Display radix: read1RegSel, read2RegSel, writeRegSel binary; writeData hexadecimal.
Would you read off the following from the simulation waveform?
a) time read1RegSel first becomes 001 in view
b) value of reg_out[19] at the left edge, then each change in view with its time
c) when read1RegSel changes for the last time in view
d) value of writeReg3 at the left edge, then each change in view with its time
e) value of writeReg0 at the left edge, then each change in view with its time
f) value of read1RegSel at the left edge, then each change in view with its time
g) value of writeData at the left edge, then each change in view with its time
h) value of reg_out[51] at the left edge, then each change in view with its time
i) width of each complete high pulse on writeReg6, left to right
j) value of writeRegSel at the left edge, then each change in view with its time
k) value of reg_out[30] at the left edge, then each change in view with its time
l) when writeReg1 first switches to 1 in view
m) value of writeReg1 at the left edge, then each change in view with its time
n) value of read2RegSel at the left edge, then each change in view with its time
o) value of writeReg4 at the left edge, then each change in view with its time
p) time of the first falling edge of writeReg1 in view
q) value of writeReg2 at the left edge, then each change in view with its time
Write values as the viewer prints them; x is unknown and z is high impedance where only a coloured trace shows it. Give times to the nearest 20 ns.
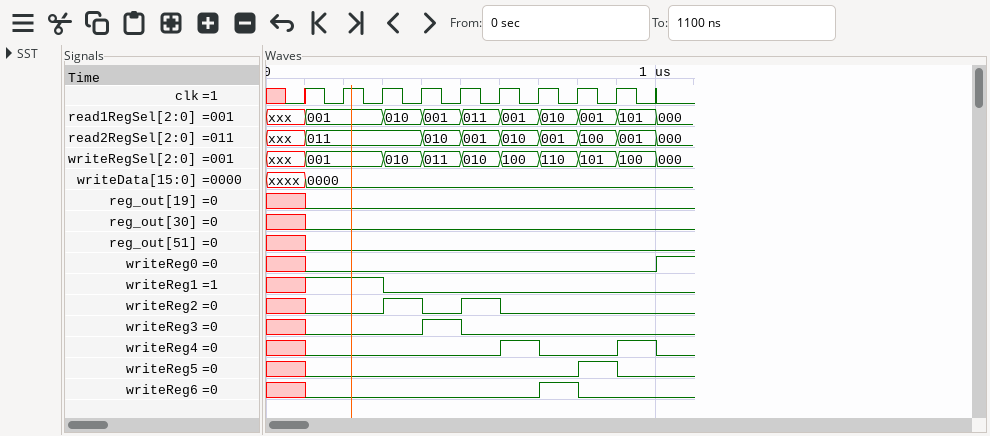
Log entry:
100 ns
x, 0 at 100 ns
1000 ns
x, 0 at 100 ns, 1 at 400 ns, 0 at 500 ns
x, 0 at 100 ns, 1 at 1000 ns
xxx, 001 at 100 ns, 010 at 300 ns, 001 at 400 ns, 011 at 500 ns, 001 at 600 ns, 010 at 700 ns, 001 at 800 ns, 101 at 900 ns, 000 at 1000 ns
xxxx, 0000 at 100 ns
x, 0 at 100 ns
100 ns
xxx, 001 at 100 ns, 010 at 300 ns, 011 at 400 ns, 010 at 500 ns, 100 at 600 ns, 110 at 700 ns, 101 at 800 ns, 100 at 900 ns, 000 at 1000 ns
x, 0 at 100 ns
100 ns
x, 1 at 100 ns, 0 at 300 ns
xxx, 011 at 100 ns, 010 at 400 ns, 001 at 500 ns, 010 at 600 ns, 001 at 700 ns, 100 at 800 ns, 001 at 900 ns, 000 at 1000 ns
x, 0 at 100 ns, 1 at 600 ns, 0 at 700 ns, 1 at 900 ns, 0 at 1000 ns
300 ns
x, 0 at 100 ns, 1 at 300 ns, 0 at 400 ns, 1 at 500 ns, 0 at 600 ns
